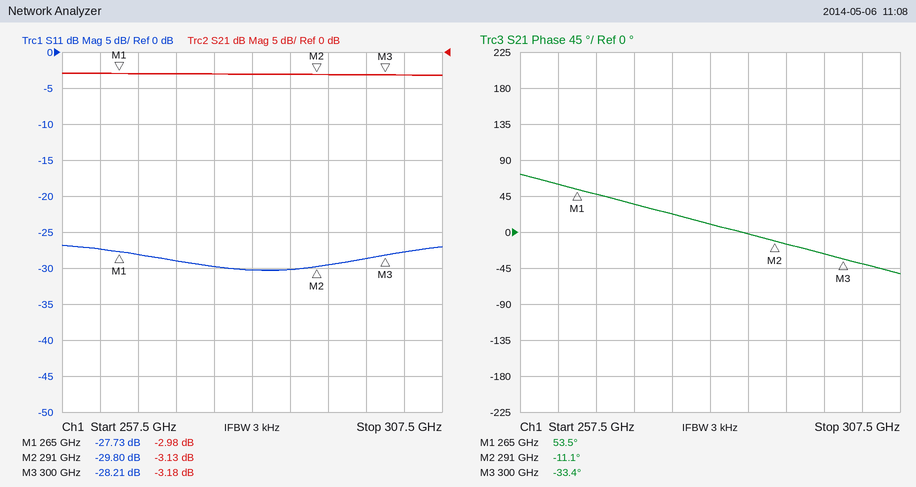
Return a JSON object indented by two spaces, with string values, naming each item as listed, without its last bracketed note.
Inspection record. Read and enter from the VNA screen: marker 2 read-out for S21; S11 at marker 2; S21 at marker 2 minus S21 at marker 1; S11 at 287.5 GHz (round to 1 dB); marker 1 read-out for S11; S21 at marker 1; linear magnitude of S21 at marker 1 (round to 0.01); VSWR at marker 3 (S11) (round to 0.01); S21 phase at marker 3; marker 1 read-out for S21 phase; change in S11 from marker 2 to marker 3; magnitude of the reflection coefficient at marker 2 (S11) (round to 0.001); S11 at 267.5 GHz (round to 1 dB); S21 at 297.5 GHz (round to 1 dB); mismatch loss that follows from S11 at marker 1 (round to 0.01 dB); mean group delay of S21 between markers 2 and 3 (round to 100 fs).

{
  "marker 2 read-out for S21": "-3.13 dB",
  "S11 at marker 2": "-29.80 dB",
  "S21 at marker 2 minus S21 at marker 1": "-0.15 dB",
  "S11 at 287.5 GHz": "-30 dB",
  "marker 1 read-out for S11": "-27.73 dB",
  "S21 at marker 1": "-2.98 dB",
  "linear magnitude of S21 at marker 1": "0.71",
  "VSWR at marker 3 (S11)": "1.08",
  "S21 phase at marker 3": "-33.4°",
  "marker 1 read-out for S21 phase": "53.5°",
  "change in S11 from marker 2 to marker 3": "1.59 dB",
  "magnitude of the reflection coefficient at marker 2 (S11)": "0.032",
  "S11 at 267.5 GHz": "-28 dB",
  "S21 at 297.5 GHz": "-3 dB",
  "mismatch loss that follows from S11 at marker 1": "0.01 dB",
  "mean group delay of S21 between markers 2 and 3": "6.9 ps"
}
